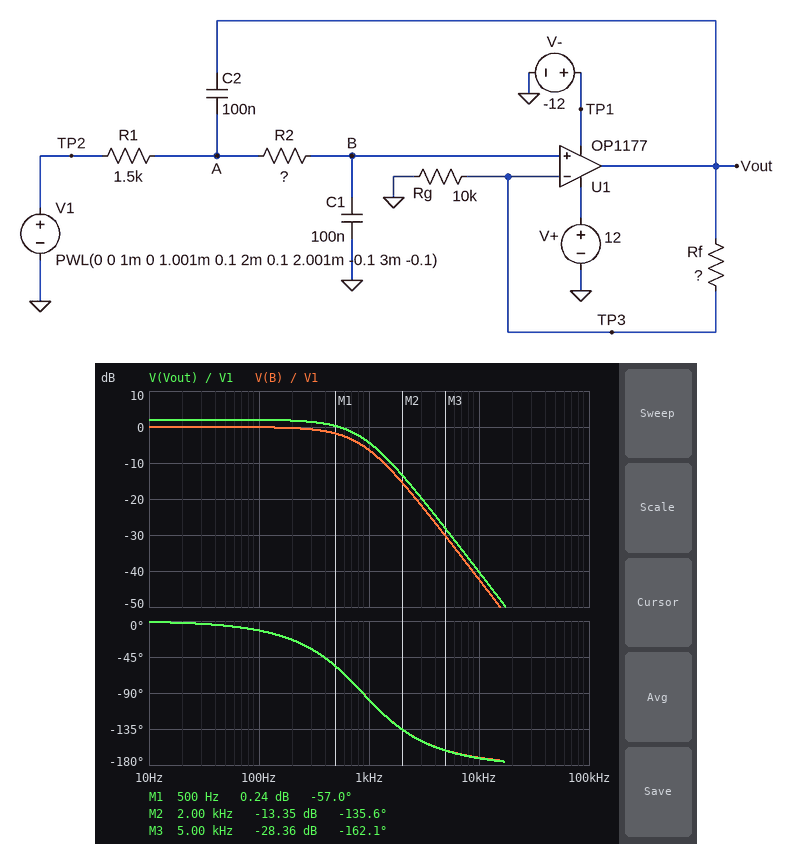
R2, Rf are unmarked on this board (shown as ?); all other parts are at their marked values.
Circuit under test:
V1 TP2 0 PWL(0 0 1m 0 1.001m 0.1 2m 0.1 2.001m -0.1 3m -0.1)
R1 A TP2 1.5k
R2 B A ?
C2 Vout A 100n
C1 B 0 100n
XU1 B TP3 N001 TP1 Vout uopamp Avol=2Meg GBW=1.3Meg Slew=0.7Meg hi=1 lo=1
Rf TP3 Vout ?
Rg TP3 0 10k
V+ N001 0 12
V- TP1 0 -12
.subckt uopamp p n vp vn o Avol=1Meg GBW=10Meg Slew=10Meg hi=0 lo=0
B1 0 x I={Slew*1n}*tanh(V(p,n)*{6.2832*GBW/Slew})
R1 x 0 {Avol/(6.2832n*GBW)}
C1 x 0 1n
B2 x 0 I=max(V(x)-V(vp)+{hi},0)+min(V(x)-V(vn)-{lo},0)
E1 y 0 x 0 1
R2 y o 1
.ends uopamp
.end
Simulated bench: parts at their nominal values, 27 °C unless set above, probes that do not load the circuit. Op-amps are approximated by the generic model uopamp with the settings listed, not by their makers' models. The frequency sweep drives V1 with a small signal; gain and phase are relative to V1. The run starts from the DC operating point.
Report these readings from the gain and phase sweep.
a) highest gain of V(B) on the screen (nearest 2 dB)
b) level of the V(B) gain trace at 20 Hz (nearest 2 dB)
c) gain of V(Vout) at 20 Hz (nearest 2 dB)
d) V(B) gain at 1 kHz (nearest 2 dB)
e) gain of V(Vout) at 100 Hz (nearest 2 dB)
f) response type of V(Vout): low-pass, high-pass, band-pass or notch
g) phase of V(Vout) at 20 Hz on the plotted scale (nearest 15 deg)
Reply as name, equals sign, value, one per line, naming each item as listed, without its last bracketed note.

highest gain of V(B) on the screen = 0 dB
level of the V(B) gain trace at 20 Hz = 0 dB
gain of V(Vout) at 20 Hz = 2 dB
V(B) gain at 1 kHz = -6 dB
gain of V(Vout) at 100 Hz = 2 dB
response type of V(Vout): low-pass, high-pass, band-pass or notch = low-pass
phase of V(Vout) at 20 Hz on the plotted scale = 0 deg
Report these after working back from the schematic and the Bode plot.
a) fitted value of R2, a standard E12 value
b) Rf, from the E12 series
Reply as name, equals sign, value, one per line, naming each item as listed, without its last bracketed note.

fitted value of R2, a standard E12 value = 2.2 kΩ
Rf, from the E12 series = 2.7 kΩ
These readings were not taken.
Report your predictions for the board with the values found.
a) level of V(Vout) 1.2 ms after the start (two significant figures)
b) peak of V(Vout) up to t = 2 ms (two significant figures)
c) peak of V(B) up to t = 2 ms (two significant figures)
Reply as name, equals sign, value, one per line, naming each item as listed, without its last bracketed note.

level of V(Vout) 1.2 ms after the start = 40 mV
peak of V(Vout) up to t = 2 ms = 130 mV
peak of V(B) up to t = 2 ms = 99 mV
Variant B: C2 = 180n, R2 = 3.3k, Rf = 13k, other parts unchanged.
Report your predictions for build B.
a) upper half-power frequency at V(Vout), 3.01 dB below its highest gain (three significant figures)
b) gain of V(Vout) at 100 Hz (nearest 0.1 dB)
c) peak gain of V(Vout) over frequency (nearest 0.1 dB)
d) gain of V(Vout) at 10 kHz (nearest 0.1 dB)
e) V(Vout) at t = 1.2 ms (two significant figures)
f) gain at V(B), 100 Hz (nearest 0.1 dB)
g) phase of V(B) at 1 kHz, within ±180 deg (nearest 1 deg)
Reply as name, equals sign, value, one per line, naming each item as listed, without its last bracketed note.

upper half-power frequency at V(Vout), 3.01 dB below its highest gain = 614 Hz
gain of V(Vout) at 100 Hz = 7.5 dB
peak gain of V(Vout) over frequency = 14.7 dB
gain of V(Vout) at 10 kHz = -43.7 dB
V(Vout) at t = 1.2 ms = 45 mV
gain at V(B), 100 Hz = 0.3 dB
phase of V(B) at 1 kHz, within ±180 deg = -162 deg
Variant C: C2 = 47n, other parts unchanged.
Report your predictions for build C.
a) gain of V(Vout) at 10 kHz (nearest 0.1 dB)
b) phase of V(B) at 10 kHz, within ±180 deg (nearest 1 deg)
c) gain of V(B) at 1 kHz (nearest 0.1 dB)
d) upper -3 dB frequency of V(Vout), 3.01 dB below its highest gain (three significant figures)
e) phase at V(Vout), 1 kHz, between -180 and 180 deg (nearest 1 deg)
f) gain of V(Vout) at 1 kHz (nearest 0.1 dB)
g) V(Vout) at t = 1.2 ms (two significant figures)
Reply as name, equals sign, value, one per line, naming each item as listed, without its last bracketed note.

gain of V(Vout) at 10 kHz = -34.1 dB
phase of V(B) at 10 kHz, within ±180 deg = -160 deg
gain of V(B) at 1 kHz = -7.0 dB
upper -3 dB frequency of V(Vout), 3.01 dB below its highest gain = 517 Hz
phase at V(Vout), 1 kHz, between -180 and 180 deg = -80 deg
gain of V(Vout) at 1 kHz = -4.9 dB
V(Vout) at t = 1.2 ms = 49 mV
